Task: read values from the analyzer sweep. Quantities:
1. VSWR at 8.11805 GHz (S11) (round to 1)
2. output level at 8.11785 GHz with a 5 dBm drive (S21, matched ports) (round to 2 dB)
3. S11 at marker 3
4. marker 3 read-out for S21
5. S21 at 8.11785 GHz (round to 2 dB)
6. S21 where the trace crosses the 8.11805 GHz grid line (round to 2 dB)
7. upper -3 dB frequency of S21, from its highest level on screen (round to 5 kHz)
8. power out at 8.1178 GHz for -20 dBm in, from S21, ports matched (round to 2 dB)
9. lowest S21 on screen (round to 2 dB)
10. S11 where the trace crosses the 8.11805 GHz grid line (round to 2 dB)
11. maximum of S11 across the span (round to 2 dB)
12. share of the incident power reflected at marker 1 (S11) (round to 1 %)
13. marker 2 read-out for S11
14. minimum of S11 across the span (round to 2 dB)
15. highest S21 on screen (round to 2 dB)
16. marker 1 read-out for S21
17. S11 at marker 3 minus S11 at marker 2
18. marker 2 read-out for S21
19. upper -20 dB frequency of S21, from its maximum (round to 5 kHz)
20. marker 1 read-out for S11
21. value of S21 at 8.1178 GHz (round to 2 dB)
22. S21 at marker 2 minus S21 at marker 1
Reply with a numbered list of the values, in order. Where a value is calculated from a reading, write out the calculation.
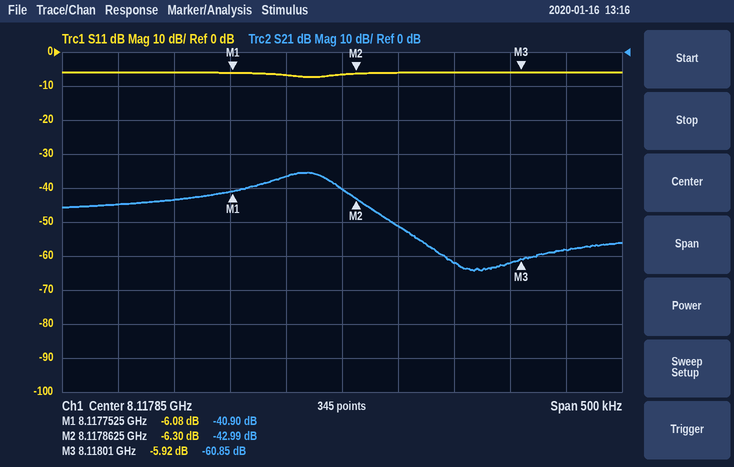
1. |Γ| = 10^(-6/20) = 0.5012; VSWR = (1 + 0.5012)/(1 − 0.5012) ≈ 3
2. 5 dBm + (-40 dB) = -36 dBm
3. -5.92 dB
4. -60.85 dB
5. -40 dB
6. -58 dB
7. 8.117840 GHz
8. -20 dBm + (-36 dB) = -56 dBm
9. -64 dB
10. -6 dB
11. -6 dB
12. 10^(-6.08/10) ≈ 25 %
13. -6.30 dB
14. -8 dB
15. -36 dB
16. -40.90 dB
17. -5.92 − (-6.3) = 0.38 dB
18. -42.99 dB
19. 8.117920 GHz
20. -6.08 dB
21. -36 dB
22. -42.99 − (-40.9) = -2.09 dB
